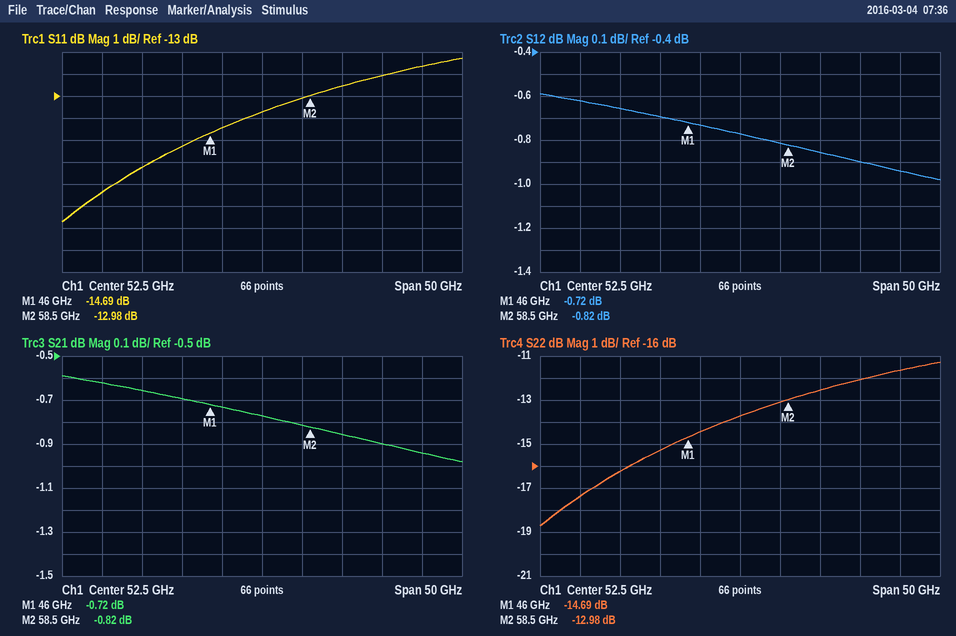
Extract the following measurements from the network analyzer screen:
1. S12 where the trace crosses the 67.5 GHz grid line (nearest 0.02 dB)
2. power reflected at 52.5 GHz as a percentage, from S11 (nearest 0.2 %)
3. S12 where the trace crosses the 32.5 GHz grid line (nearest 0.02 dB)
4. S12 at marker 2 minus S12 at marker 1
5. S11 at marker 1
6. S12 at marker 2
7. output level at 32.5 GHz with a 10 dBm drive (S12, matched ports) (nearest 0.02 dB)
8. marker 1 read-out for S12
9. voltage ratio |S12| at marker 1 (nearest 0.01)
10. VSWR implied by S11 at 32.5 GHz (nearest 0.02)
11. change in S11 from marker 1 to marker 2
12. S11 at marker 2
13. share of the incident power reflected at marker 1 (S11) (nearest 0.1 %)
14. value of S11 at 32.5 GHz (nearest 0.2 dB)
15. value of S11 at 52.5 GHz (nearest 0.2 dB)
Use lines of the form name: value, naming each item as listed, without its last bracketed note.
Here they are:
S12 where the trace crosses the 67.5 GHz grid line: -0.90 dB
power reflected at 52.5 GHz as a percentage, from S11: 4.2 %
S12 where the trace crosses the 32.5 GHz grid line: -0.62 dB
S12 at marker 2 minus S12 at marker 1: -0.10 dB
S11 at marker 1: -14.69 dB
S12 at marker 2: -0.82 dB
output level at 32.5 GHz with a 10 dBm drive (S12, matched ports): 9.38 dBm
marker 1 read-out for S12: -0.72 dB
voltage ratio |S12| at marker 1: 0.92
VSWR implied by S11 at 32.5 GHz: 1.32
change in S11 from marker 1 to marker 2: 1.71 dB
S11 at marker 2: -12.98 dB
share of the incident power reflected at marker 1 (S11): 3.4 %
value of S11 at 32.5 GHz: -17.4 dB
value of S11 at 52.5 GHz: -13.8 dB
